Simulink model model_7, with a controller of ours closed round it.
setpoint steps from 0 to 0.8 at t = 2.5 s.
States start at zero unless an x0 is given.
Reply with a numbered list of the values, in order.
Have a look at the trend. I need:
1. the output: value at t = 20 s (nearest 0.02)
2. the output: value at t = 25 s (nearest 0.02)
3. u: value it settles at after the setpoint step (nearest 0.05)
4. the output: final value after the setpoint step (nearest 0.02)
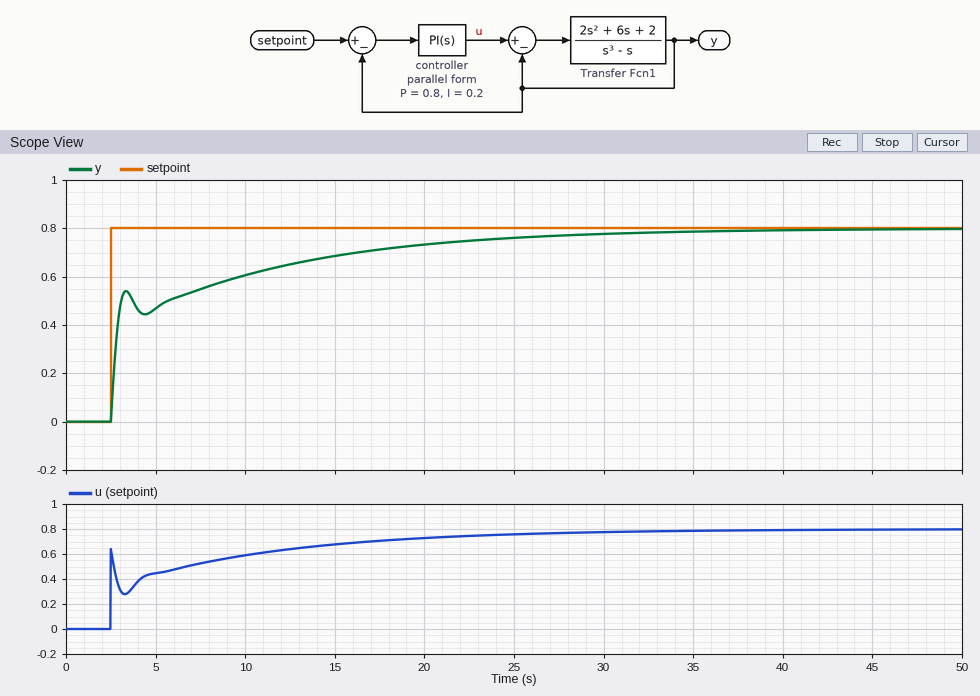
1. 0.74
2. 0.76
3. 0.80
4. 0.80
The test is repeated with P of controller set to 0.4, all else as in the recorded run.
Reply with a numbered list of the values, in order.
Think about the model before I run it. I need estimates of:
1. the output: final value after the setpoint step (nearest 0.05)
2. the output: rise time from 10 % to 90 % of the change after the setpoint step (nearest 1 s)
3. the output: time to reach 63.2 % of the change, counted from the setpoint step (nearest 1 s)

1. 0.80
2. 14 s
3. 4 s
